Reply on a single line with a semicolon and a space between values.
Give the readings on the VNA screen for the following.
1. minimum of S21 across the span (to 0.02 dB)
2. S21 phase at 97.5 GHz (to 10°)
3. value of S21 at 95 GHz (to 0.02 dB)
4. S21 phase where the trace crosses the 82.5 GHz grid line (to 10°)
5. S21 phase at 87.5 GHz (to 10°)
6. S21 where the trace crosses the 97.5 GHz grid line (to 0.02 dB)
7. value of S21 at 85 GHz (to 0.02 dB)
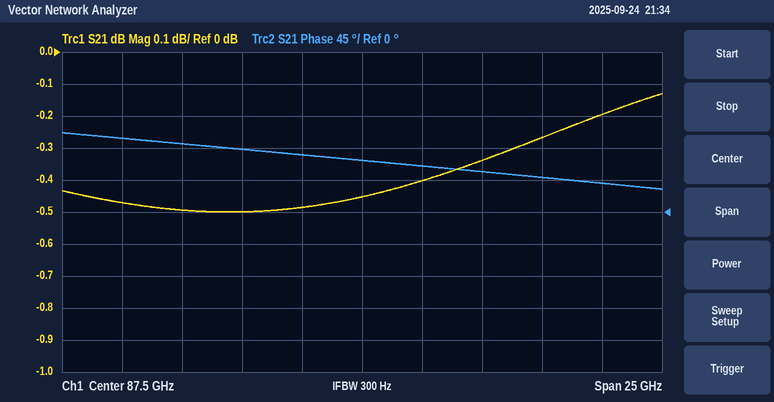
-0.50 dB; 40°; -0.26 dB; 90°; 70°; -0.20 dB; -0.48 dB
